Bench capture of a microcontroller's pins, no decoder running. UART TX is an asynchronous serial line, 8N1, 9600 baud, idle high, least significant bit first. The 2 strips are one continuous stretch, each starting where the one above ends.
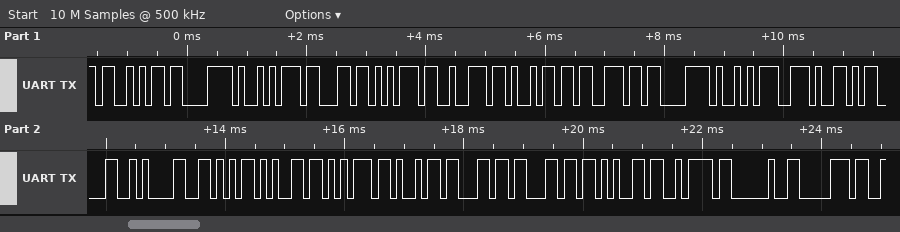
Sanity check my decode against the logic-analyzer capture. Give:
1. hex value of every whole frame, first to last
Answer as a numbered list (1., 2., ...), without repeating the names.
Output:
1. 0x53 0xC3 0xA9 0x63 0x75 0x72 0x69 0x73 0xC3 0xA9 0x2E 0x0D 0x0A 0x56 0x65 0x75 0x69 0x6C 0x6C 0x65 0x7A 0x20 0x70
